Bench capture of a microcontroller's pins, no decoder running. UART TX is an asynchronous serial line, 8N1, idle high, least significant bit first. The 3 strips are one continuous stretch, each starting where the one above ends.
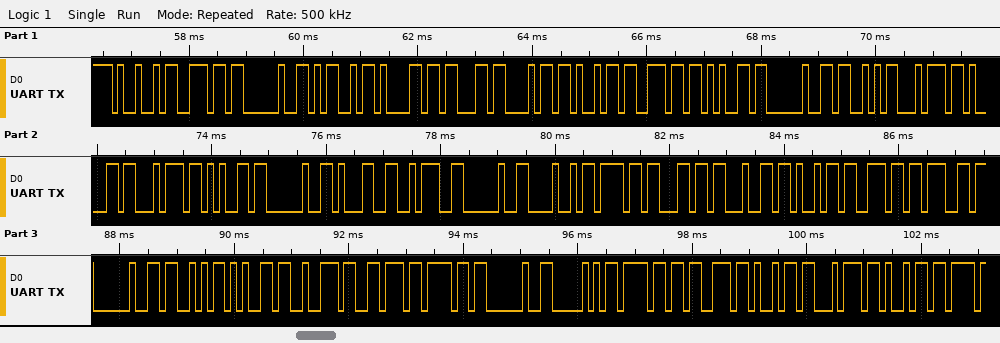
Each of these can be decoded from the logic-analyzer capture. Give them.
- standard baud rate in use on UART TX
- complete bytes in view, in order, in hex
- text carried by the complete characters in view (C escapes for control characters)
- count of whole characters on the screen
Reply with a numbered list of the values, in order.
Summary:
1. 9600 baud
2. 49 6E 20 4D 61 63 68 69 6E 65 20 53 74 61 74 65 20 31 3A 20 48 6F 6C 64 69 6E 67 20 53 65 72 76 6F 20 50 6F 73 69 74 69
3. "In Machine State 1: Holding Servo Positi"
4. 40
